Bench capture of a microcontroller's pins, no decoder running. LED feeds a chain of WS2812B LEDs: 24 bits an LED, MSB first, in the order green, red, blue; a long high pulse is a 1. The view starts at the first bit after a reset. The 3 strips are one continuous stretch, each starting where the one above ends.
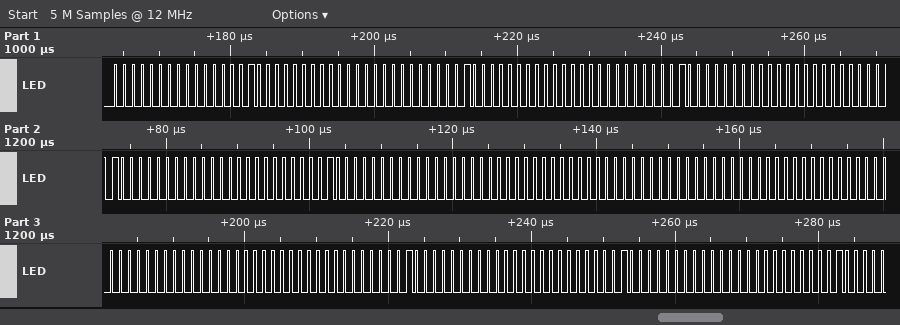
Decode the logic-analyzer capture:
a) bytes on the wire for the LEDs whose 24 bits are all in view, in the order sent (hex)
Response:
00 01 00 00 01 00 00 01 00 00 01 00 00 01 00 00 00 00 00 00 00 00 00 00 00 01 00 00 01 00
